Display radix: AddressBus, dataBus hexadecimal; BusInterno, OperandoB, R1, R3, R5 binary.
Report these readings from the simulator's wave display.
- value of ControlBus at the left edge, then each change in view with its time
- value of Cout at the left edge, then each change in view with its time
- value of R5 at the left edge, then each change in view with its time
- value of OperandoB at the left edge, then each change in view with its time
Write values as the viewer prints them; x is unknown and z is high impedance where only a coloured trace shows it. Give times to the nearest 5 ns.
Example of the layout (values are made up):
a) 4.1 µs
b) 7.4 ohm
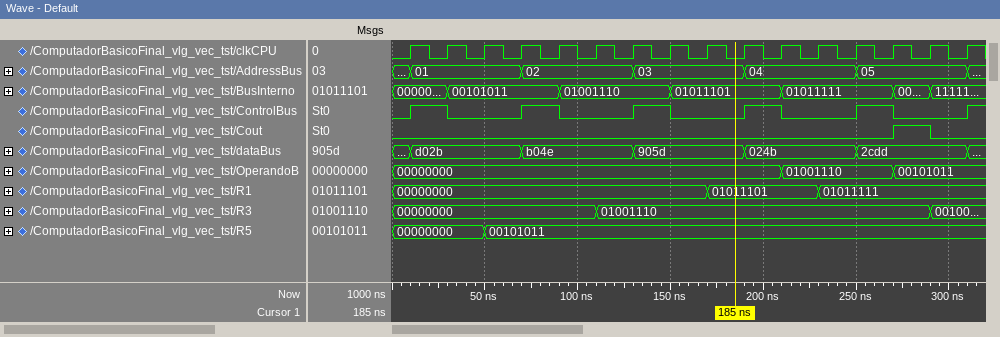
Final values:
a) 0, 1 at 10 ns, 0 at 30 ns, 1 at 70 ns, 0 at 90 ns, 1 at 130 ns, 0 at 150 ns, 1 at 190 ns, 0 at 210 ns, 1 at 250 ns, 0 at 270 ns, 1 at 310 ns
b) 0, 1 at 270 ns, 0 at 290 ns
c) 00000000, 00101011 at 50 ns
d) 00000000, 01001110 at 210 ns, 00101011 at 270 ns
